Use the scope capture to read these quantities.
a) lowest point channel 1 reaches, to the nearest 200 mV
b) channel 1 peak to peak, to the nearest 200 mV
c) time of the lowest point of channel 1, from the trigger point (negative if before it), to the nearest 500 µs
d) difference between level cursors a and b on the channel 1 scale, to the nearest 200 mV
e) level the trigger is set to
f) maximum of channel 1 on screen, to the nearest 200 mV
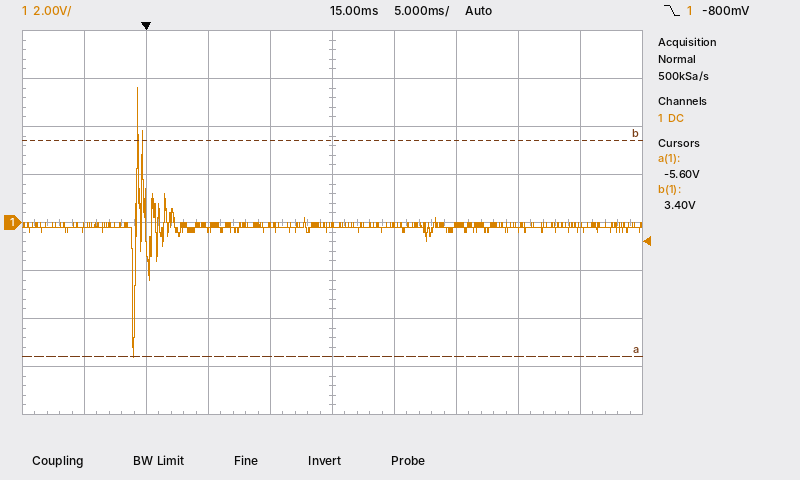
-5.6 V
11.2 V
-1.0 ms
9.0 V
-800 mV
5.6 V
